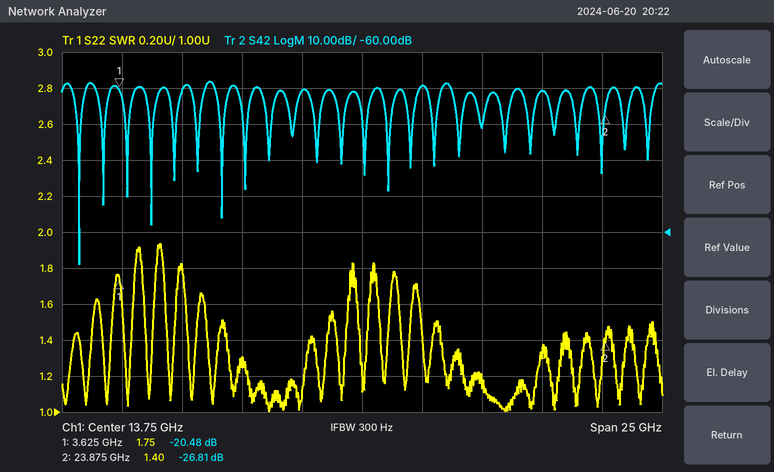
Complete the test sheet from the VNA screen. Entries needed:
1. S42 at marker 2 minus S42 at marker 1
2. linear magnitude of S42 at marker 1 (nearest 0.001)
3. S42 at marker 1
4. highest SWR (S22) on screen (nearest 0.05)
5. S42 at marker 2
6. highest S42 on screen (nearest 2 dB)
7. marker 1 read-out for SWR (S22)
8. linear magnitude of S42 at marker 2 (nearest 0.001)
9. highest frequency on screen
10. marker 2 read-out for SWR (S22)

-6.33 dB
0.095
-20.48 dB
1.95
-26.81 dB
-18 dB
1.75
0.046
26.25 GHz
1.40
